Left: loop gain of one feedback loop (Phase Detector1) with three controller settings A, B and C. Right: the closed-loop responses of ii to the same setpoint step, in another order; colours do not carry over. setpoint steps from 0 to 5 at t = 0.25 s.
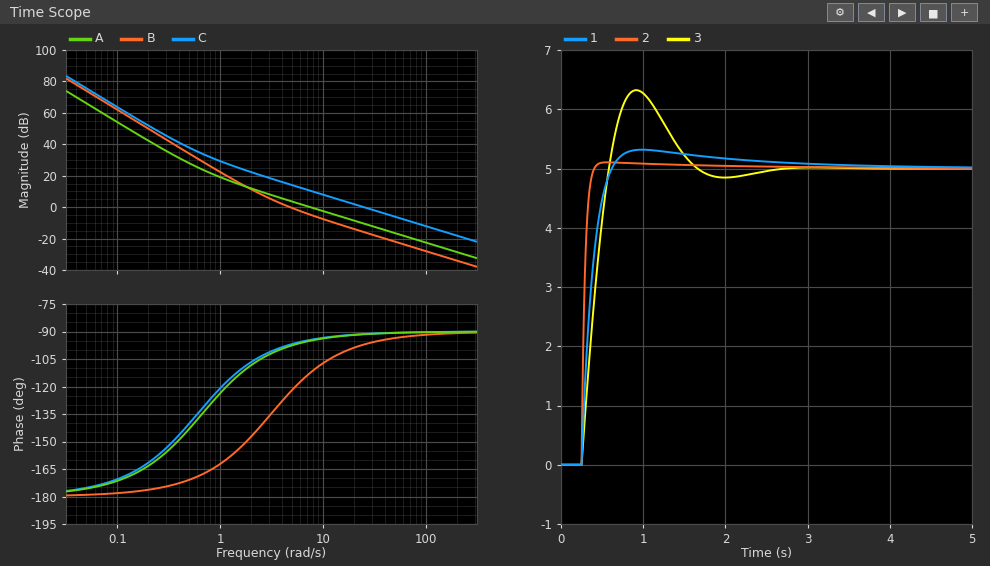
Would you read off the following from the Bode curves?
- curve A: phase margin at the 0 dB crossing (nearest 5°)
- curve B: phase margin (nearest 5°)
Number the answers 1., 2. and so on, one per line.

1. 85°
2. 55°
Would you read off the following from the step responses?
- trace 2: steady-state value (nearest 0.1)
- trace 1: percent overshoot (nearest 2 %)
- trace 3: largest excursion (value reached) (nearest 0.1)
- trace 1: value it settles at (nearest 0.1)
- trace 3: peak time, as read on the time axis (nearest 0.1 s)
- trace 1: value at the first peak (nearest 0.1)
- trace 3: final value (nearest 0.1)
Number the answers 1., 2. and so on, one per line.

1. 5.0
2. 6 %
3. 6.3
4. 5.0
5. 0.9 s
6. 5.3
7. 5.0
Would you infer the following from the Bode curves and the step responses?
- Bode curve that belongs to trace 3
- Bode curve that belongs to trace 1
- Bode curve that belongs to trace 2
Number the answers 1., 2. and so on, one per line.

1. B
2. A
3. C
